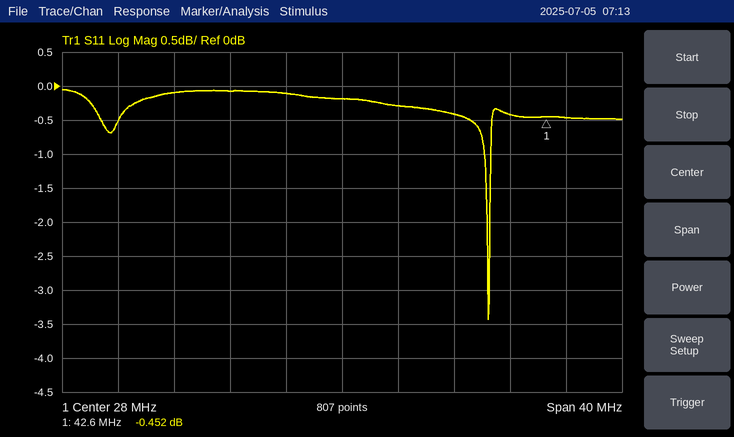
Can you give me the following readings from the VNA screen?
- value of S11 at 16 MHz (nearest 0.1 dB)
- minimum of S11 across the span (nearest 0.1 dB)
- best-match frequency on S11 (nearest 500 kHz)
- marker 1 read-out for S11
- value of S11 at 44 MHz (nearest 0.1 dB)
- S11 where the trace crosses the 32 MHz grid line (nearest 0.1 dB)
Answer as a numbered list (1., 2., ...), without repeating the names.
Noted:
1. -0.1 dB
2. -3.4 dB
3. 38.5 MHz
4. -0.452 dB
5. -0.5 dB
6. -0.3 dB
